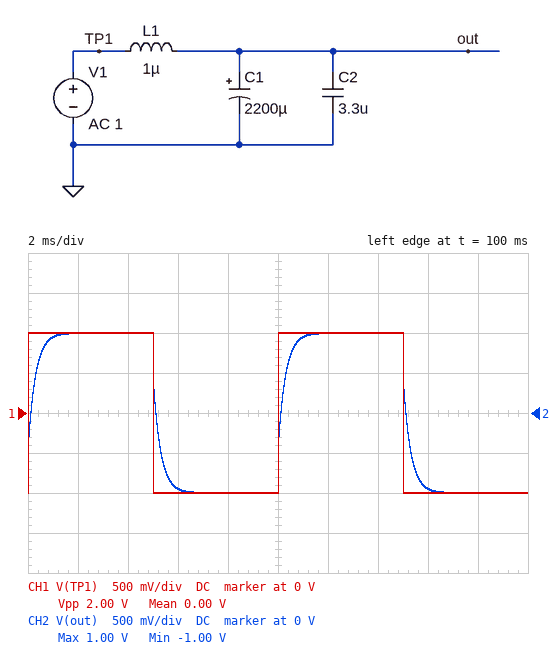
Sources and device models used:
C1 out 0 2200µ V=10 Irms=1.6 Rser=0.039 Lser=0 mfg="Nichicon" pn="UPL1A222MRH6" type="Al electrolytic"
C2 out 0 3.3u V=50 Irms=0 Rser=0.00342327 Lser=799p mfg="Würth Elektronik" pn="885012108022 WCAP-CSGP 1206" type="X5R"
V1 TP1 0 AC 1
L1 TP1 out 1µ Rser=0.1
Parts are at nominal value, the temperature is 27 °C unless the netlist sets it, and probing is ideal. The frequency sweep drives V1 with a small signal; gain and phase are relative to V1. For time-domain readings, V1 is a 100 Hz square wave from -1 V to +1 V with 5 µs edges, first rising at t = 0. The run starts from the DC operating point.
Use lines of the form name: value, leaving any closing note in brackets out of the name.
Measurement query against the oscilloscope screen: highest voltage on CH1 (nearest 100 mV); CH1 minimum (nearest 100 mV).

highest voltage on CH1: 1.0 V
CH1 minimum: -1.0 V
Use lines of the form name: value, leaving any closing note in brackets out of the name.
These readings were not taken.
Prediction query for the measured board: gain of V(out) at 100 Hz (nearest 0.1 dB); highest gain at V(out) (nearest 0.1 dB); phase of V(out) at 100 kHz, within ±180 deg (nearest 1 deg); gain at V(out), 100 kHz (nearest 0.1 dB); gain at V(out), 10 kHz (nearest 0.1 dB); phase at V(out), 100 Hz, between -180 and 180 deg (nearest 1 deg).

gain of V(out) at 100 Hz: -0.1 dB
highest gain at V(out): 0 dB
phase of V(out) at 100 kHz, within ±180 deg: -83 deg
gain at V(out), 100 kHz: -24.3 dB
gain at V(out), 10 kHz: -11.5 dB
phase at V(out), 100 Hz, between -180 and 180 deg: -8 deg
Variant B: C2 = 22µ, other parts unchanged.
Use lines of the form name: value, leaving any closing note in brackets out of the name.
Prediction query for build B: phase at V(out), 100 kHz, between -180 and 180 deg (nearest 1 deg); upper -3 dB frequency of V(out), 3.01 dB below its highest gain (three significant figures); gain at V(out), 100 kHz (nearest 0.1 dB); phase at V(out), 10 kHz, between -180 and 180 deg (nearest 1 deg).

phase at V(out), 100 kHz, between -180 and 180 deg: -107 deg
upper -3 dB frequency of V(out), 3.01 dB below its highest gain: 580 Hz
gain at V(out), 100 kHz: -25.5 dB
phase at V(out), 10 kHz, between -180 and 180 deg: -35 deg
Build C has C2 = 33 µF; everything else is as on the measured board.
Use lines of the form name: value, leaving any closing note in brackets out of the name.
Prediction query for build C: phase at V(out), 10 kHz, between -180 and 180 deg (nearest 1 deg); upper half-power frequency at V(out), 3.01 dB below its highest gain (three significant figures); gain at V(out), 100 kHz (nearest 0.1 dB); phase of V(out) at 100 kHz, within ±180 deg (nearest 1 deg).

phase at V(out), 10 kHz, between -180 and 180 deg: -36 deg
upper half-power frequency at V(out), 3.01 dB below its highest gain: 578 Hz
gain at V(out), 100 kHz: -26.6 dB
phase of V(out) at 100 kHz, within ±180 deg: -117 deg
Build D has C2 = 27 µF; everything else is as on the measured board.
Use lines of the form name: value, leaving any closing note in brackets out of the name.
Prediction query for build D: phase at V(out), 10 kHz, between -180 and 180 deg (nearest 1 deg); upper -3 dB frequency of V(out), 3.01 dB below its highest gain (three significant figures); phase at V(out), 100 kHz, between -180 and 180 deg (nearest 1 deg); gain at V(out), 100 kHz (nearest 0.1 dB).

phase at V(out), 10 kHz, between -180 and 180 deg: -35 deg
upper -3 dB frequency of V(out), 3.01 dB below its highest gain: 579 Hz
phase at V(out), 100 kHz, between -180 and 180 deg: -112 deg
gain at V(out), 100 kHz: -26.0 dB
